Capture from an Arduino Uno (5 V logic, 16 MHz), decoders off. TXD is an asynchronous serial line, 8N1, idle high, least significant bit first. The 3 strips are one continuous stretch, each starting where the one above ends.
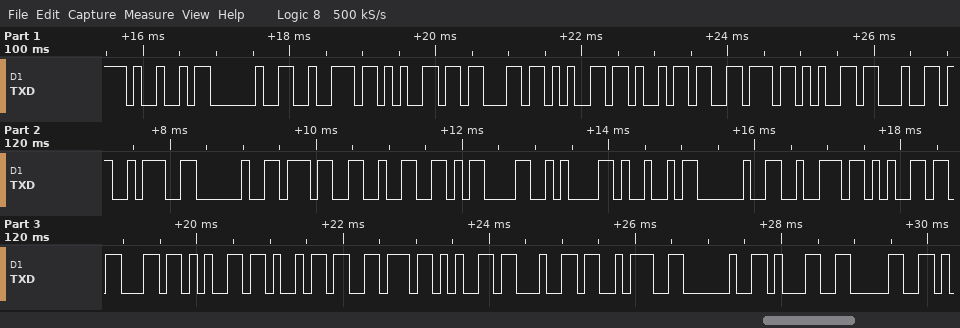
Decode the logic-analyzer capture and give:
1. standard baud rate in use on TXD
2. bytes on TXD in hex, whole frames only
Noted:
9600 baud
49 20 72 65 63 65 69 76 65 64 3A 20 37 32 0D 0A 49 20 72 65 63 65 69 76 65 64 3A 20 31 30
